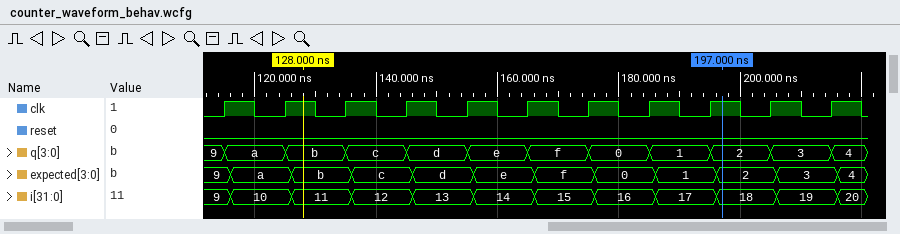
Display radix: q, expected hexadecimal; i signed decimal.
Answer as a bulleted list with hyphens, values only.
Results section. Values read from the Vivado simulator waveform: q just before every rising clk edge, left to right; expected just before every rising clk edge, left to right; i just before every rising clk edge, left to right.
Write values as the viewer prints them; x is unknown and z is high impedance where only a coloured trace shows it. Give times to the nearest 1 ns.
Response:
- 9, a, b, c, d, e, f, 0, 1, 2, 3
- 9, a, b, c, d, e, f, 0, 1, 2, 3
- 9, 10, 11, 12, 13, 14, 15, 16, 17, 18, 19
